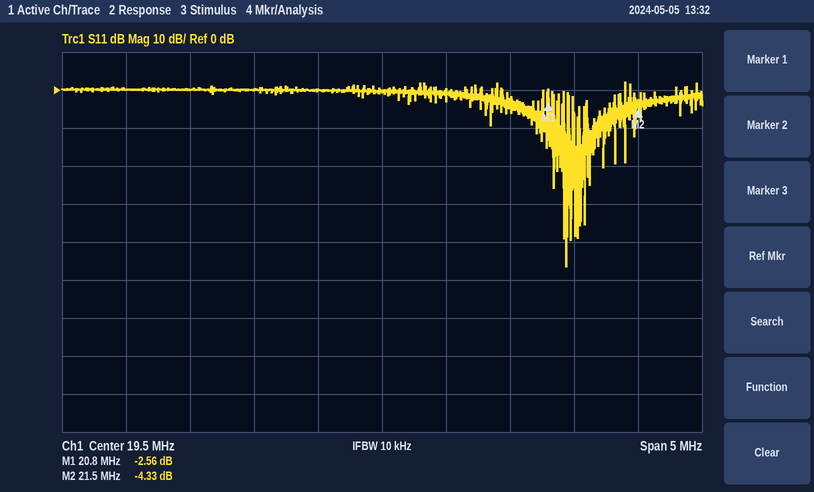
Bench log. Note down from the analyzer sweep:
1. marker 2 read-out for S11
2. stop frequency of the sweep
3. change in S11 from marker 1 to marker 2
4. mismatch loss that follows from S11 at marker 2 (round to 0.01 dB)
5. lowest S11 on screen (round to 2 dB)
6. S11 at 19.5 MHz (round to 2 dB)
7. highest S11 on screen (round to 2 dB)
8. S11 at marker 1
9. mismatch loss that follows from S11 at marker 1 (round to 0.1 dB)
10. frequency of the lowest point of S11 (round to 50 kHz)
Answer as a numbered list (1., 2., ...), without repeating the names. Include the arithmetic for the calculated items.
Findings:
1. -4.33 dB
2. 22 MHz
3. -4.33 − (-2.56) = -1.77 dB
4. −10 log10(1 − 10^(-4.33/10)) ≈ 2.00 dB
5. -46 dB
6. 0 dB
7. 2 dB
8. -2.56 dB
9. −10 log10(1 − 10^(-2.56/10)) ≈ 3.5 dB
10. 20.95 MHz
